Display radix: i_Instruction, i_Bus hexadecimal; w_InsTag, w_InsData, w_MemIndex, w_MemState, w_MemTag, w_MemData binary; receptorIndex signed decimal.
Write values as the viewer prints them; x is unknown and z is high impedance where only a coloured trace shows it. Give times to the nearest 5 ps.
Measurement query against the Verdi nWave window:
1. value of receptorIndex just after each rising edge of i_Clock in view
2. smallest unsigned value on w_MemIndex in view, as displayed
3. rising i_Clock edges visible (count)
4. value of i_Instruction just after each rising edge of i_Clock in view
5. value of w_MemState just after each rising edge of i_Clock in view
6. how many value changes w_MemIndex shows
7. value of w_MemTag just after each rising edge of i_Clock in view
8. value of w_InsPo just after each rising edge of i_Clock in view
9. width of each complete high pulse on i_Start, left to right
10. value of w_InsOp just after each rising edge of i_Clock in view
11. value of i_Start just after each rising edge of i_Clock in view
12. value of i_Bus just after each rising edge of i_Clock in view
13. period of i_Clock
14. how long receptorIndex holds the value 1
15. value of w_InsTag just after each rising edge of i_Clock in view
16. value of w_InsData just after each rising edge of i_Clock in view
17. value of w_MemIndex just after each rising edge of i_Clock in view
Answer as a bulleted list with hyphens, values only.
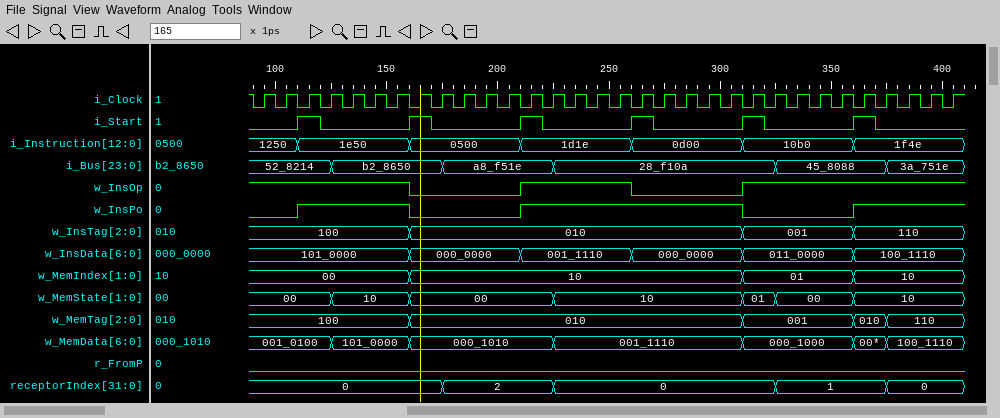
- 0, 0, 0, 0, 0, 0, 0, 0, 2, 2, 2, 2, 2, 0, 0, 0, 0, 0, 0, 0, 0, 0, 0, 1, 1, 1, 1, 1, 0, 0, 0, 0
- 00
- 32
- 1250, 1250, 1e50, 1e50, 1e50, 1e50, 1e50, 0500, 0500, 0500, 0500, 0500, 1d1e, 1d1e, 1d1e, 1d1e, 1d1e, 0d00, 0d00, 0d00, 0d00, 0d00, 10b0, 10b0, 10b0, 10b0, 10b0, 1f4e, 1f4e, 1f4e, 1f4e, 1f4e
- 00, 00, 00, 10, 10, 10, 10, 00, 00, 00, 00, 00, 00, 10, 10, 10, 10, 10, 10, 10, 10, 10, 01, 00, 00, 00, 00, 10, 10, 10, 10, 10
- 3
- 100, 100, 100, 100, 100, 100, 100, 010, 010, 010, 010, 010, 010, 010, 010, 010, 010, 010, 010, 010, 010, 010, 001, 001, 001, 001, 001, 010, 110, 110, 110, 110
- 0 0 1 1 1 1 1 0 0 0 0 0 1 1 1 1 1 1 1 1 1 1 0 0 0 0 0 1 1 1 1 1
- 10 ps, 10 ps, 10 ps, 10 ps, 10 ps, 10 ps
- 1 1 1 1 1 1 1 0 0 0 0 0 1 1 1 1 1 0 0 0 0 0 1 1 1 1 1 1 1 1 1 1
- 0 0 1 0 0 0 0 1 0 0 0 0 1 0 0 0 0 1 0 0 0 0 1 0 0 0 0 1 0 0 0 0
- 52_8214, 52_8214, 52_8214, b2_8650, b2_8650, b2_8650, b2_8650, b2_8650, a8_f51e, a8_f51e, a8_f51e, a8_f51e, a8_f51e, 28_f10a, 28_f10a, 28_f10a, 28_f10a, 28_f10a, 28_f10a, 28_f10a, 28_f10a, 28_f10a, 28_f10a, 45_8088, 45_8088, 45_8088, 45_8088, 45_8088, 3a_751e, 3a_751e, 3a_751e, 3a_751e
- 10 ps
- 50 ps
- 100, 100, 100, 100, 100, 100, 100, 010, 010, 010, 010, 010, 010, 010, 010, 010, 010, 010, 010, 010, 010, 010, 001, 001, 001, 001, 001, 110, 110, 110, 110, 110
- 101_0000, 101_0000, 101_0000, 101_0000, 101_0000, 101_0000, 101_0000, 000_0000, 000_0000, 000_0000, 000_0000, 000_0000, 001_1110, 001_1110, 001_1110, 001_1110, 001_1110, 000_0000, 000_0000, 000_0000, 000_0000, 000_0000, 011_0000, 011_0000, 011_0000, 011_0000, 011_0000, 100_1110, 100_1110, 100_1110, 100_1110, 100_1110
- 00, 00, 00, 00, 00, 00, 00, 10, 10, 10, 10, 10, 10, 10, 10, 10, 10, 10, 10, 10, 10, 10, 01, 01, 01, 01, 01, 10, 10, 10, 10, 10
